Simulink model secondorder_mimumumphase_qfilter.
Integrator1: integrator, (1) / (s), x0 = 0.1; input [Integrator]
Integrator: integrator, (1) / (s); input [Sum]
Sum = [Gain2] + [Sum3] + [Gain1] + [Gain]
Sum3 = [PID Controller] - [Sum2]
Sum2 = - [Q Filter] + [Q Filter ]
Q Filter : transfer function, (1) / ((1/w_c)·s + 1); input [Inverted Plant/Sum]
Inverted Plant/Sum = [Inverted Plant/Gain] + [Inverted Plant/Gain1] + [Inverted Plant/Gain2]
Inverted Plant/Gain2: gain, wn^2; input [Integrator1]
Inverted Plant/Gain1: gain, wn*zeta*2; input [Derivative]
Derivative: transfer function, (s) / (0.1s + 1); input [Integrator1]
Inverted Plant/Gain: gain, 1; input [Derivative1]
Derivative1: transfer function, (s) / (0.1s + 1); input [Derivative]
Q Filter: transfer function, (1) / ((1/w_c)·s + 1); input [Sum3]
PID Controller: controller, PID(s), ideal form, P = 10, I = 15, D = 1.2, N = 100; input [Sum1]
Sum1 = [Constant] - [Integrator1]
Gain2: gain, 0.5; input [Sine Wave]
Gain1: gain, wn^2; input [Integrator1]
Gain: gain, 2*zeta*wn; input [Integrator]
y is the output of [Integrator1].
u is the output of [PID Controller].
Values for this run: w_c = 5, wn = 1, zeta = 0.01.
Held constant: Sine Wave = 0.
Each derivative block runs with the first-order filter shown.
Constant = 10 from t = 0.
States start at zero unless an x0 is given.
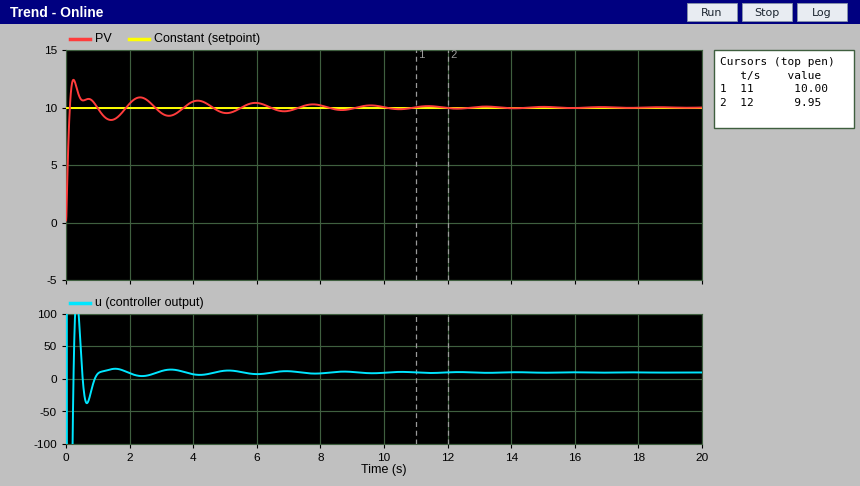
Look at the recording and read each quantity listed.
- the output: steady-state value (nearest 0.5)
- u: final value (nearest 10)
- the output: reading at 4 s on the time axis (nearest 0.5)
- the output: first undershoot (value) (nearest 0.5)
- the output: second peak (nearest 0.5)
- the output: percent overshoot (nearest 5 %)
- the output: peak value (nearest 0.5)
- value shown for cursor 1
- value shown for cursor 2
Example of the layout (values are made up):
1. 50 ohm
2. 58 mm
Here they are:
1. 10.0
2. 10
3. 10.5
4. 9.0
5. 11.0
6. 25 %
7. 12.5
8. 10.00
9. 9.95
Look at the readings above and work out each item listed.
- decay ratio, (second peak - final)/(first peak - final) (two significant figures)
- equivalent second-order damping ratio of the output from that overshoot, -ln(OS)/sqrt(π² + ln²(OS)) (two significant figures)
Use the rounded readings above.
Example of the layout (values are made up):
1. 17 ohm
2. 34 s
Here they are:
1. 0.40
2. 0.40
